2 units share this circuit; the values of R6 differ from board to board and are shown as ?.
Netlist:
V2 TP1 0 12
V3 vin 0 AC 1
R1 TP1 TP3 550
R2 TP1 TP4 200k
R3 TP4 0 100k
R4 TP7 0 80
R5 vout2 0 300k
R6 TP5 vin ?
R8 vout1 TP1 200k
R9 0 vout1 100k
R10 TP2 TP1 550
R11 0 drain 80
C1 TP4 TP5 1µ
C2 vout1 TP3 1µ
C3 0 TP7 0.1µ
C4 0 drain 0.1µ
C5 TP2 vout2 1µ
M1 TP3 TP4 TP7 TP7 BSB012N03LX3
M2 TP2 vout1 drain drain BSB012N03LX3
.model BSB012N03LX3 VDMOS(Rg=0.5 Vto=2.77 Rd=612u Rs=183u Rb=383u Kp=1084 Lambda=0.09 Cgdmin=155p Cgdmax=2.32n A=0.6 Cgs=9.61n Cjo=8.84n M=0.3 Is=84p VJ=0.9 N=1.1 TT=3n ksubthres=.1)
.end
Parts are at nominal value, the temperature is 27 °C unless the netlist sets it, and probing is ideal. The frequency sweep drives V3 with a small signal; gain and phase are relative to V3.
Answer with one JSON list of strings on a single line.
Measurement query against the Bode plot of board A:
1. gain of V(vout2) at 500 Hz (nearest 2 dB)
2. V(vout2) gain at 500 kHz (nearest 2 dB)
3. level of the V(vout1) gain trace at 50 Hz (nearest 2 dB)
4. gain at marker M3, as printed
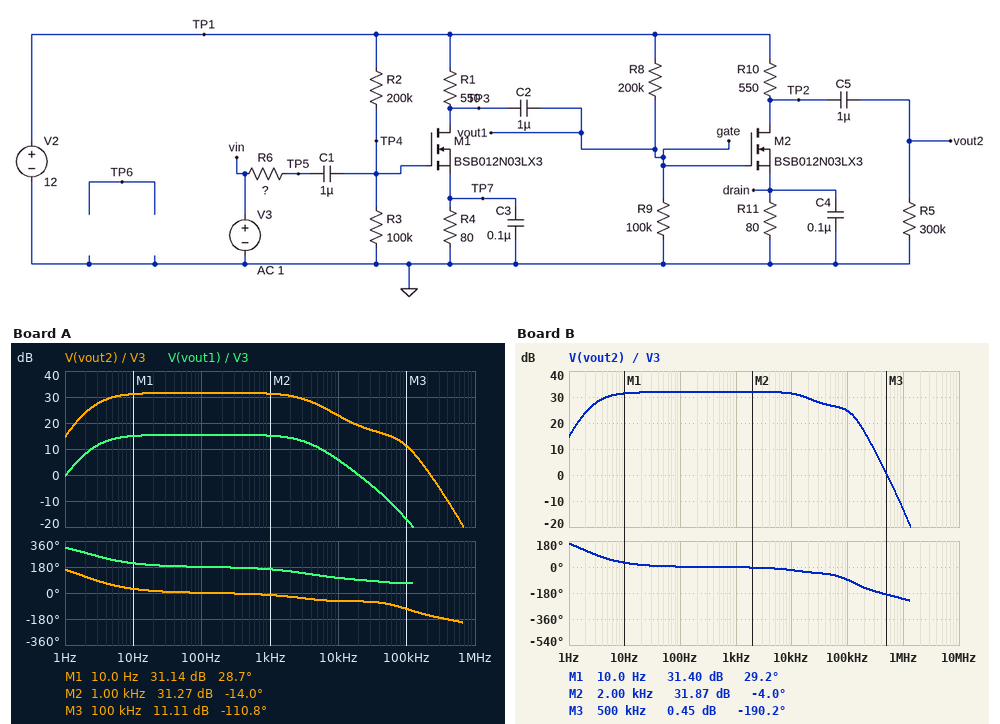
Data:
["32 dB", "-14 dB", "16 dB", "11.11 dB"]
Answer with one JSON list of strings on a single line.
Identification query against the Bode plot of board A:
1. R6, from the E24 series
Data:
["2.7 kΩ"]
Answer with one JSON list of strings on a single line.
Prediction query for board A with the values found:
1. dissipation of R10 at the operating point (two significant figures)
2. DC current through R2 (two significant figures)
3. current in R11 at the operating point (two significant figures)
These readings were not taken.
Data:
["200 mW", "40 µA", "19 mA"]
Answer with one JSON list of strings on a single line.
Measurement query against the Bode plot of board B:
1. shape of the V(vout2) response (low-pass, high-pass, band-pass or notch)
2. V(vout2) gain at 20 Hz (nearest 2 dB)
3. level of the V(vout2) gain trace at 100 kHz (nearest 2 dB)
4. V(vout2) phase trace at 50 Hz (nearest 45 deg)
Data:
["band-pass", "32 dB", "24 dB", "0 deg"]
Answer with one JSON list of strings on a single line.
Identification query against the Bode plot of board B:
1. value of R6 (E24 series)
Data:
["510 Ω"]
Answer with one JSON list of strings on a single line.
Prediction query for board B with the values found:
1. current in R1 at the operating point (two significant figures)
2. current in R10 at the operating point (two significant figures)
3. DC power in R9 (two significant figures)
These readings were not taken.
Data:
["19 mA", "19 mA", "160 µW"]
